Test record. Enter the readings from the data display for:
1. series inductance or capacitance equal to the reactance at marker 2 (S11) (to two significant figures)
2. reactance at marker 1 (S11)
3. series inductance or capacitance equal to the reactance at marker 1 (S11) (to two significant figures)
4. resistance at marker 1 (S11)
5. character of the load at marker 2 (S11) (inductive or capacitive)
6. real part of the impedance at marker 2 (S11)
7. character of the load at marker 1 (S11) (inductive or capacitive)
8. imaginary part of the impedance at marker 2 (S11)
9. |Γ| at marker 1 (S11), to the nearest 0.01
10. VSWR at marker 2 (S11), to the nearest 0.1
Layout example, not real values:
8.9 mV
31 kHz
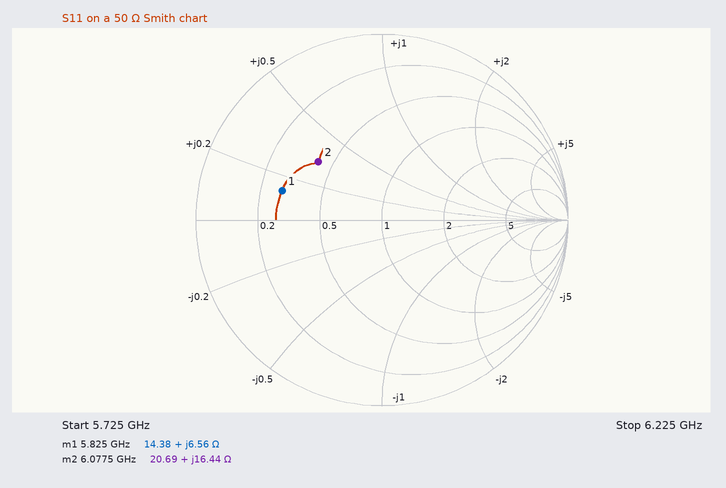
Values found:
430 pH
+6.56 Ω
180 pH
14.38 Ω
inductive
20.69 Ω
inductive
+16.44 Ω
0.56
2.7
